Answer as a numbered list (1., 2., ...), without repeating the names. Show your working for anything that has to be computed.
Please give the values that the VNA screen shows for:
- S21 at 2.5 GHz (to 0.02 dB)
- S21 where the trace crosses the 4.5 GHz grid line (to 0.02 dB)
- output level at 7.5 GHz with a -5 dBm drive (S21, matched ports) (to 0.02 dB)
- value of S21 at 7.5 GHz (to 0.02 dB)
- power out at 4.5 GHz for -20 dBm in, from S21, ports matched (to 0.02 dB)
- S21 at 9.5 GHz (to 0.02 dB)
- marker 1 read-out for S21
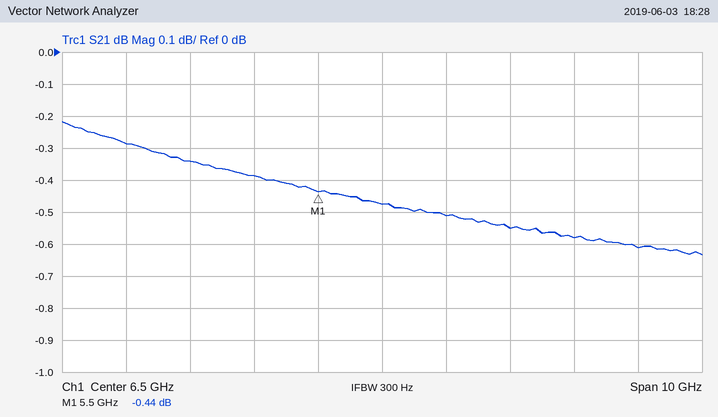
1. -0.28 dB
2. -0.38 dB
3. -5 dBm + (-0.52 dB) = -5.52 dBm
4. -0.52 dB
5. -20 dBm + (-0.38 dB) = -20.38 dBm
6. -0.58 dB
7. -0.44 dB
